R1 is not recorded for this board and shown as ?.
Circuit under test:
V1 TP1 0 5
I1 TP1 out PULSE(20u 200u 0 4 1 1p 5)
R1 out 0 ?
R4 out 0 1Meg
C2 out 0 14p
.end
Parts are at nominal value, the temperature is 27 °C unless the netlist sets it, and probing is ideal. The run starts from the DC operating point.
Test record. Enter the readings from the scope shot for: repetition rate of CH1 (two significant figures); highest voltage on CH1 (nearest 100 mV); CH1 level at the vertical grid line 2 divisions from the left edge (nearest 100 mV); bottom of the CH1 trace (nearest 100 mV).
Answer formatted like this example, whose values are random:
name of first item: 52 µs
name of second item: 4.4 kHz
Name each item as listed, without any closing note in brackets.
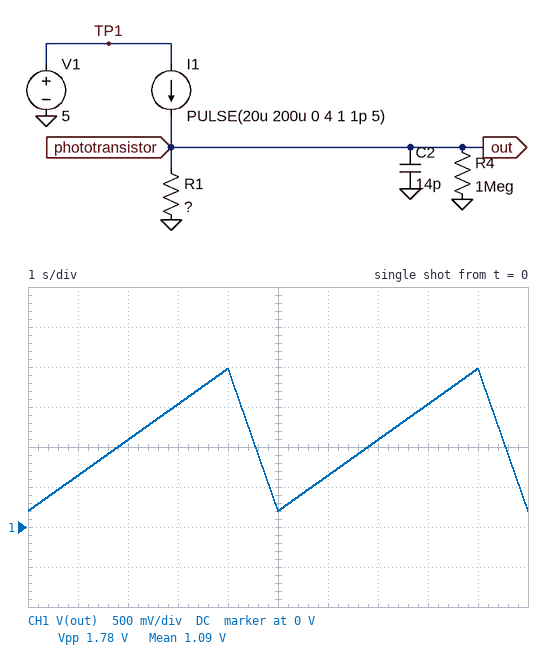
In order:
repetition rate of CH1: 200 mHz
highest voltage on CH1: 2.0 V
CH1 level at the vertical grid line 2 divisions from the left edge: 1.1 V
bottom of the CH1 trace: 200 mV
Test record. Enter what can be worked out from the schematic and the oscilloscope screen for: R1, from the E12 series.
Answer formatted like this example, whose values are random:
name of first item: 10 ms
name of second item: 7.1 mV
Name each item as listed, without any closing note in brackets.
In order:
R1, from the E12 series: 10 kΩ
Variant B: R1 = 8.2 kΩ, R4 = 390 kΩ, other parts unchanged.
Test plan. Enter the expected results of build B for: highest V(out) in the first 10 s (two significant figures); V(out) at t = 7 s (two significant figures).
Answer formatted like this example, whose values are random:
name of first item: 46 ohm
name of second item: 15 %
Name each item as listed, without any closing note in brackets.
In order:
highest V(out) in the first 10 s: 1.6 V
V(out) at t = 7 s: 880 mV
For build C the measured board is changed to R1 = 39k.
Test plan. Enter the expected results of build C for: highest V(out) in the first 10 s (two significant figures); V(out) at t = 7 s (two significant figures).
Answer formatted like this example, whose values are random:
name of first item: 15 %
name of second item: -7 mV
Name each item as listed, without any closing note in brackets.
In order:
highest V(out) in the first 10 s: 7.5 V
V(out) at t = 7 s: 4.1 V
